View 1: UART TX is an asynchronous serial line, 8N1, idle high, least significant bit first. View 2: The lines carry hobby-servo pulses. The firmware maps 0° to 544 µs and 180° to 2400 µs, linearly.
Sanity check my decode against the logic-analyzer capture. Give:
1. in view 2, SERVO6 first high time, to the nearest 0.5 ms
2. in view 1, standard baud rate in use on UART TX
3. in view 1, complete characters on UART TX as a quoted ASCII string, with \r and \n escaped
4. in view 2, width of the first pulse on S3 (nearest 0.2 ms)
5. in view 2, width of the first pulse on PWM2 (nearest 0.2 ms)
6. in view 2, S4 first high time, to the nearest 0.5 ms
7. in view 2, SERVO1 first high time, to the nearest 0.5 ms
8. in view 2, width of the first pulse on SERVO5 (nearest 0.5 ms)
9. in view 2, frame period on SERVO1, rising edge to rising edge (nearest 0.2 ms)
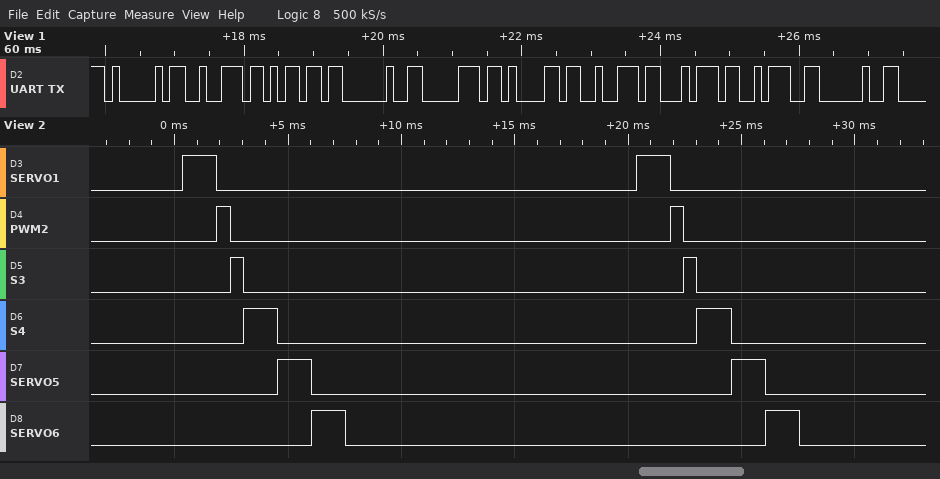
1.5 ms
9600 baud
"Arm part: "
0.6 ms
0.6 ms
1.5 ms
1.5 ms
1.5 ms
20.0 ms
